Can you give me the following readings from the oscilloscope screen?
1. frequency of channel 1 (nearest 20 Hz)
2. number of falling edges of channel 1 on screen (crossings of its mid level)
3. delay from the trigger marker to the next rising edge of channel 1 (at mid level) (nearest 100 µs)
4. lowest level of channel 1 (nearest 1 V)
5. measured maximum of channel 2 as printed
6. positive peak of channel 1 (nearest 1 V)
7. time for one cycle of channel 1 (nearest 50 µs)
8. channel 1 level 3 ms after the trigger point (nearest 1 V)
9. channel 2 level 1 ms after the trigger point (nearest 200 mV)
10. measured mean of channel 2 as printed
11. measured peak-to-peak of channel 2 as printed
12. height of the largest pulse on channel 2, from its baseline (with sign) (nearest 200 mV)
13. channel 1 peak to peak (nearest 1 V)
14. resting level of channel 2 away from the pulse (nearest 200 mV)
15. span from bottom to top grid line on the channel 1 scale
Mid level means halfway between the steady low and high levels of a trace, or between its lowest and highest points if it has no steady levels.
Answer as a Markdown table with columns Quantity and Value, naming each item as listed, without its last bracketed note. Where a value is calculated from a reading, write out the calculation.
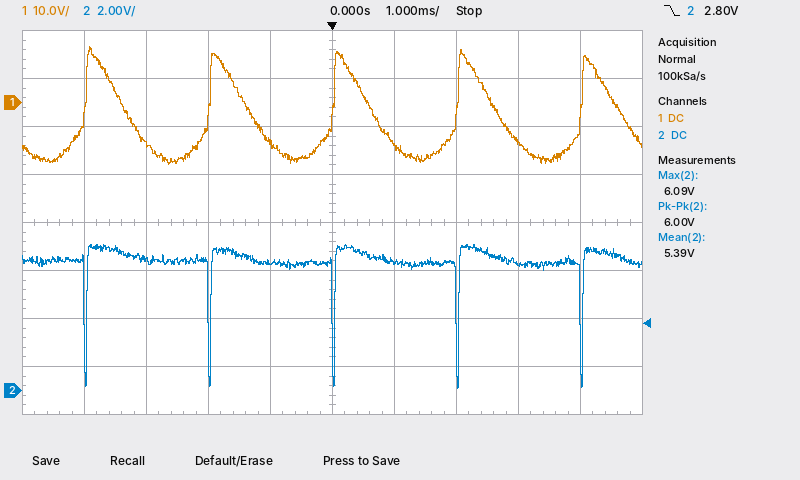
| Quantity | Value |
|---|---|
| frequency of channel 1 | 1 / 2.00 ms ≈ 500 Hz |
| number of falling edges of channel 1 on screen | 5 |
| delay from the trigger marker to the next rising edge of channel 1 (at mid level) | 2.0 ms |
| lowest level of channel 1 | -13 V |
| measured maximum of channel 2 as printed | 6.09 V |
| positive peak of channel 1 | 12 V |
| time for one cycle of channel 1 | 2.00 ms |
| channel 1 level 3 ms after the trigger point | -8 V |
| channel 2 level 1 ms after the trigger point | 5.4 V |
| measured mean of channel 2 as printed | 5.39 V |
| measured peak-to-peak of channel 2 as printed | 6.00 V |
| height of the largest pulse on channel 2, from its baseline (with sign) | -5.2 V |
| channel 1 peak to peak | 12 V − (-13 V) = 25 V |
| resting level of channel 2 away from the pulse | 5.4 V |
| span from bottom to top grid line on the channel 1 scale | 80 V |
